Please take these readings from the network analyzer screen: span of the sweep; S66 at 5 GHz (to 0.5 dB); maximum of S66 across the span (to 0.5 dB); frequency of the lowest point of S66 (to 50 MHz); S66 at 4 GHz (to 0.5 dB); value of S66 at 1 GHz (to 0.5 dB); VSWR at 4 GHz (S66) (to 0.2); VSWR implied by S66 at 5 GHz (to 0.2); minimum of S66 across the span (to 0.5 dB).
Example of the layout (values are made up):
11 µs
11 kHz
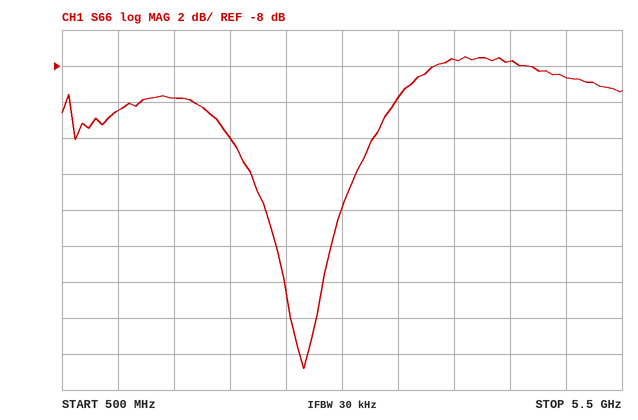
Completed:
5 GHz
-8.5 dB
-7.5 dB
2.65 GHz
-7.5 dB
-10.5 dB
2.4
2.2
-25.0 dB
